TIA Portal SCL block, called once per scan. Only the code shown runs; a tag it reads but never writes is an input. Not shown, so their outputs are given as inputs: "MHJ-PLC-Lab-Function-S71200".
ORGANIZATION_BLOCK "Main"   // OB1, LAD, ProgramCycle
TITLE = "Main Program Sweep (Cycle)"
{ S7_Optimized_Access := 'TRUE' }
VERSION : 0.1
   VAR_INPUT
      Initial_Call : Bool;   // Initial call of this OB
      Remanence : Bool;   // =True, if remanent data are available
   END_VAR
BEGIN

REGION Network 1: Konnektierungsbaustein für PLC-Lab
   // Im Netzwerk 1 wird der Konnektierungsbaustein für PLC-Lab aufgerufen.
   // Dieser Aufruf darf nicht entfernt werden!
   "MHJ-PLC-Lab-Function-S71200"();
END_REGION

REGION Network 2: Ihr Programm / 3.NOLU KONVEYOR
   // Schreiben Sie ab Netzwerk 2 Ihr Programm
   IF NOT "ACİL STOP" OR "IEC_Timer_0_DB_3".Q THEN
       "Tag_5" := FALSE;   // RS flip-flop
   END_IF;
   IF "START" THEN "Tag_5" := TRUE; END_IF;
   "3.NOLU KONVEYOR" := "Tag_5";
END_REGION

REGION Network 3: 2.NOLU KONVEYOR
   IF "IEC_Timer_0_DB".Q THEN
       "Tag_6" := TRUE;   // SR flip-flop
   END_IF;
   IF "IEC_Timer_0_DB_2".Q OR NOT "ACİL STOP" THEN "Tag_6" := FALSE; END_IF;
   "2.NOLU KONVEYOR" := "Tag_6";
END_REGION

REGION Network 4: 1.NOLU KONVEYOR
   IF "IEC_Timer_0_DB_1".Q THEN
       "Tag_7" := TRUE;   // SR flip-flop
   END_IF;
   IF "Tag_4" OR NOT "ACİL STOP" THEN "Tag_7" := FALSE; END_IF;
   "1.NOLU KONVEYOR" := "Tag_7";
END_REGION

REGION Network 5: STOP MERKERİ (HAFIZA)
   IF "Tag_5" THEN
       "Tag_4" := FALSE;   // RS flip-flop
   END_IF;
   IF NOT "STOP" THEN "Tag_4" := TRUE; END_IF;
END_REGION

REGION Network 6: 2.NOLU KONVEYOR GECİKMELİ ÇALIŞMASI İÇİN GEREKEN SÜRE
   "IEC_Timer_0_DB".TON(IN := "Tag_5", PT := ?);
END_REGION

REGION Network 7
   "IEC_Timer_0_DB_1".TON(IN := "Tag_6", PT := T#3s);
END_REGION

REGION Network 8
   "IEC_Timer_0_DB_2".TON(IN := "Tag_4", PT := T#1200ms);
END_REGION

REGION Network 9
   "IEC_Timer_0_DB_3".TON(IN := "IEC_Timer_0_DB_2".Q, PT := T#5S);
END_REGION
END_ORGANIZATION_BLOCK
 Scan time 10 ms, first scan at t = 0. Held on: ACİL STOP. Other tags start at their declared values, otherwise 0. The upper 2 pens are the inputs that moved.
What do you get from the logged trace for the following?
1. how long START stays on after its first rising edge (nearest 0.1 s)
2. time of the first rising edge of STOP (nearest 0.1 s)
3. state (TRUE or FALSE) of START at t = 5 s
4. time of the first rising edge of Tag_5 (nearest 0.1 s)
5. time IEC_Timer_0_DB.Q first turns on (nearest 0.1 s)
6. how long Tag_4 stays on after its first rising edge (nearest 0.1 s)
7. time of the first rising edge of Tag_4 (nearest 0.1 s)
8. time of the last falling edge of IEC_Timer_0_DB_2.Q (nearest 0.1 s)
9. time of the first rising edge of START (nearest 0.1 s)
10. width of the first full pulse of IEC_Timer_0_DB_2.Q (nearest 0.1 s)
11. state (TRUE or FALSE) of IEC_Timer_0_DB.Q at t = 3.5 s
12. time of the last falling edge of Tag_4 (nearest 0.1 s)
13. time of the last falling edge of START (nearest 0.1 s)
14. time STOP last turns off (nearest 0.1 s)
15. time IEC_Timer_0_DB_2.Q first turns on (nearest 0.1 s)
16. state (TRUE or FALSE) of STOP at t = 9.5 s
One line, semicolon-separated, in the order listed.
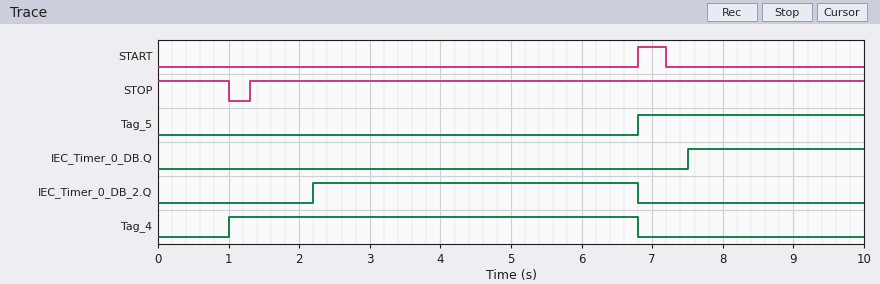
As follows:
0.4 s; 1.3 s; FALSE; 6.8 s; 7.5 s; 5.8 s; 1.0 s; 6.8 s; 6.8 s; 4.6 s; FALSE; 6.8 s; 7.2 s; 1.0 s; 2.2 s; TRUE
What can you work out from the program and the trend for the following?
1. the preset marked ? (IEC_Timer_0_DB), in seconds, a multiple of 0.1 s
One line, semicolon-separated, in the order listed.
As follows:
0.7 s
